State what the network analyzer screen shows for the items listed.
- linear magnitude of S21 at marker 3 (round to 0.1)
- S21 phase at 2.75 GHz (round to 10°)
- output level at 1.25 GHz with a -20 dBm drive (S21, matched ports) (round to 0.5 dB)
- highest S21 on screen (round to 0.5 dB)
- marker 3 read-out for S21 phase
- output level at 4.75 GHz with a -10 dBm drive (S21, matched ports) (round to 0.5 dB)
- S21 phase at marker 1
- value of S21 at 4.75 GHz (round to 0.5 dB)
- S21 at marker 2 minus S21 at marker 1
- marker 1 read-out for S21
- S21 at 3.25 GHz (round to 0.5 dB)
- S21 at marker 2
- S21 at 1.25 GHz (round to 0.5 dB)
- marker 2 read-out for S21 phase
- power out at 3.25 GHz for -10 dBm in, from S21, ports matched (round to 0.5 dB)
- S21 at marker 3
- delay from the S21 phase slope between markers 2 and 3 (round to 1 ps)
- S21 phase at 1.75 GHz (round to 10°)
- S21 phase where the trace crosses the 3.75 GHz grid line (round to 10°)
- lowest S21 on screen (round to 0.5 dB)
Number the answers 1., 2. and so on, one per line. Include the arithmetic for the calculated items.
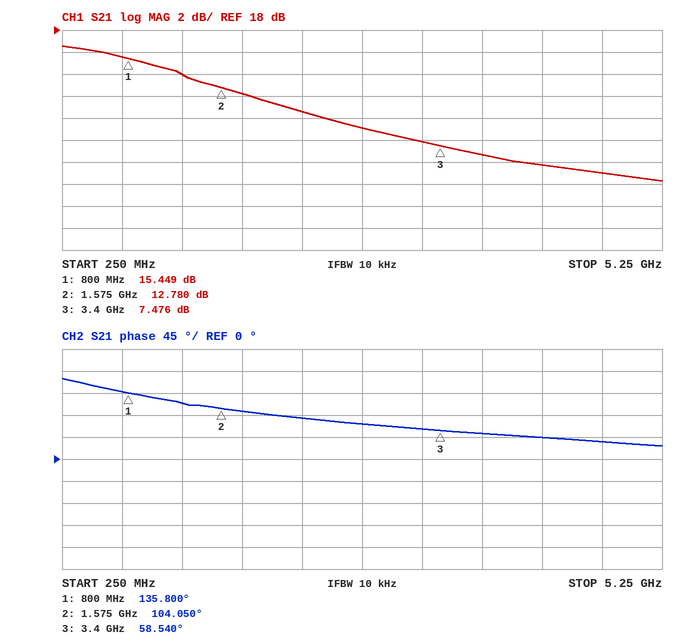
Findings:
1. 10^(7.476/20) ≈ 2.4
2. 70°
3. -20 dBm + (14.0 dB) = -6.0 dBm
4. 16.5 dB
5. 58.540°
6. -10 dBm + (5.0 dB) = -5.0 dBm
7. 135.800°
8. 5.0 dB
9. 12.78 − (15.449) = -2.669 dB
10. 15.449 dB
11. 8.0 dB
12. 12.780 dB
13. 14.0 dB
14. 104.050°
15. -10 dBm + (8.0 dB) = -2.0 dBm
16. 7.476 dB
17. −(58.54° − (104.05°))/(360° × 1.825 GHz) ≈ 69 ps
18. 100°
19. 50°
20. 4.5 dB
